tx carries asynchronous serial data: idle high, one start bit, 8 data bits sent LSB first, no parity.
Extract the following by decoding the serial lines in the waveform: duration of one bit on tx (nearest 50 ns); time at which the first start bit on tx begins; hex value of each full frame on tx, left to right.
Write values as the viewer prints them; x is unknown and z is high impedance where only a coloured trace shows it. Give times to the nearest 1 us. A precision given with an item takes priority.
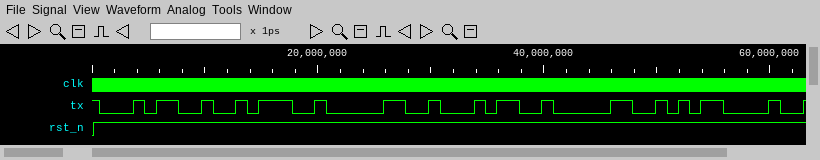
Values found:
1000 ns
1 us
34, 3A, 30, 34, 30, 0D
